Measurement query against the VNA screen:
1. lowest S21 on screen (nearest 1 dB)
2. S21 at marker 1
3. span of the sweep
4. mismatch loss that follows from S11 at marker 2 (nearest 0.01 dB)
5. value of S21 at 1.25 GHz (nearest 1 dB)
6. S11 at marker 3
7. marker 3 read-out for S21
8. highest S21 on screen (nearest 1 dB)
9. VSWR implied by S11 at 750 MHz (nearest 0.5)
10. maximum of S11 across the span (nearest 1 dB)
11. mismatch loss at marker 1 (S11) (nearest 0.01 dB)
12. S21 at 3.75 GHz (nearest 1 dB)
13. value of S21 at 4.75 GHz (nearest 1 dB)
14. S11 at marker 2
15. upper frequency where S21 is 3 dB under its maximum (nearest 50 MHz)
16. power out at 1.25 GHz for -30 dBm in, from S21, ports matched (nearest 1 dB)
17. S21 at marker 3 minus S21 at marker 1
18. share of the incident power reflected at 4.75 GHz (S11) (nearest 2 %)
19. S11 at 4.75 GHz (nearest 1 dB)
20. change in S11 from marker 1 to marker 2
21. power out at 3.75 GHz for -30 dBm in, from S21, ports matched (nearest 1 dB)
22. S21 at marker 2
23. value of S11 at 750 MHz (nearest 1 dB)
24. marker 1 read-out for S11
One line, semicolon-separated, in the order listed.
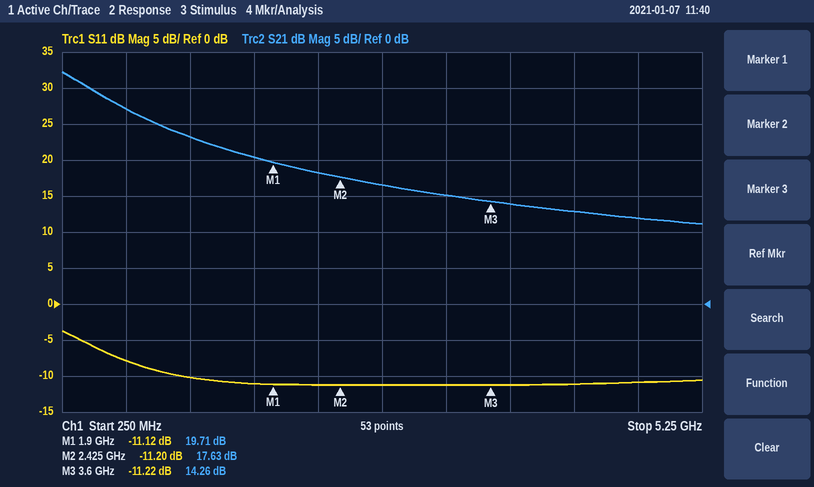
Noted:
11 dB; 19.71 dB; 5 GHz; 0.34 dB; 23 dB; -11.22 dB; 14.26 dB; 32 dB; 2.5; -4 dB; 0.35 dB; 14 dB; 12 dB; -11.20 dB; 550 MHz; -7 dBm; -5.45 dB; 8 %; -11 dB; -0.08 dB; -16 dBm; 17.63 dB; -8 dB; -11.12 dB
